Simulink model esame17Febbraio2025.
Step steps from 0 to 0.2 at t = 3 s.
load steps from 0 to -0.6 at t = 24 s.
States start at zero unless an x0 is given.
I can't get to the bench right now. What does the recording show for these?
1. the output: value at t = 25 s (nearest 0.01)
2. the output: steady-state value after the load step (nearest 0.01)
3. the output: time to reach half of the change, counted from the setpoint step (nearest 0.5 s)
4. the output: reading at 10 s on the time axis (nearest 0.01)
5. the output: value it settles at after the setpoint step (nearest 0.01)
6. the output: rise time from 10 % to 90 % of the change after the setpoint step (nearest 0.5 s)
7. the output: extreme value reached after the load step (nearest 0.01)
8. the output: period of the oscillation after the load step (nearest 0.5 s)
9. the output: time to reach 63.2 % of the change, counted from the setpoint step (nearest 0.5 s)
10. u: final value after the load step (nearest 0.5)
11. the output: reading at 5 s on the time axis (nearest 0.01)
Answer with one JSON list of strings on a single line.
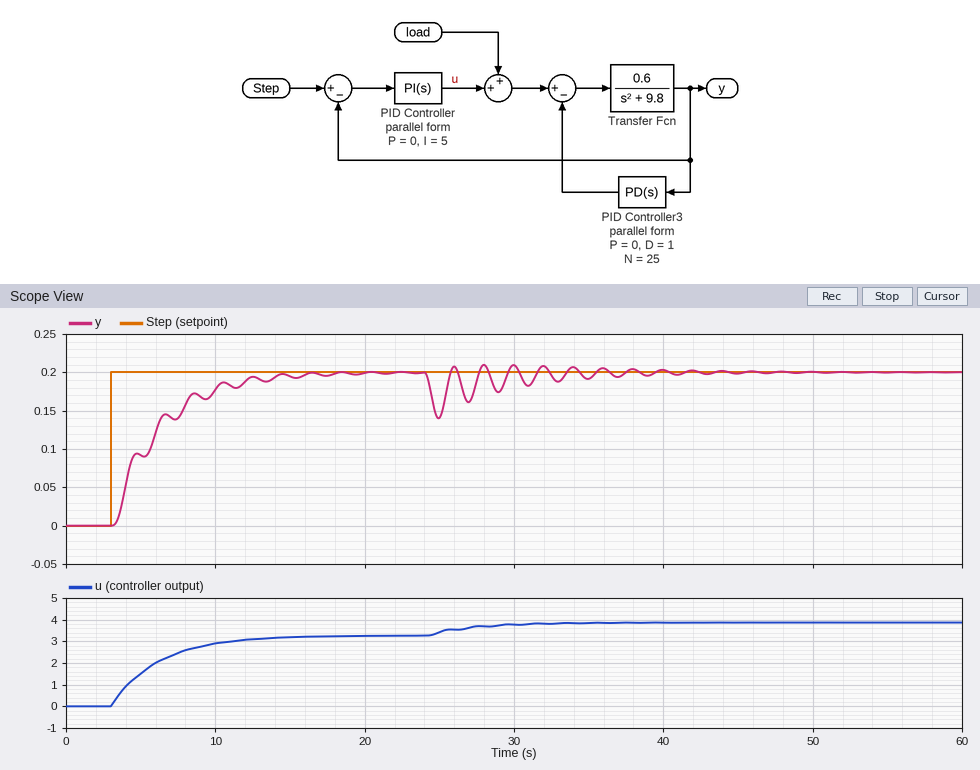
["0.14", "0.20", "2.5 s", "0.18", "0.20", "6.5 s", "0.14", "2.0 s", "3.0 s", "4.0", "0.09"]
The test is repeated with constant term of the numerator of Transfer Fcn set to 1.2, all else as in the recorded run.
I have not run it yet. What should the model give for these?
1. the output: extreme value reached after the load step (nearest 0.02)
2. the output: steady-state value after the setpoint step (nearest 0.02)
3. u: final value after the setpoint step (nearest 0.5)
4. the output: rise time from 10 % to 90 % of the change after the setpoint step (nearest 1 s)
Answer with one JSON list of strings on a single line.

["0.10", "0.20", "1.5", "3 s"]
